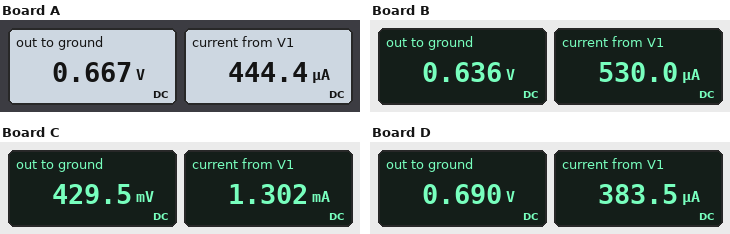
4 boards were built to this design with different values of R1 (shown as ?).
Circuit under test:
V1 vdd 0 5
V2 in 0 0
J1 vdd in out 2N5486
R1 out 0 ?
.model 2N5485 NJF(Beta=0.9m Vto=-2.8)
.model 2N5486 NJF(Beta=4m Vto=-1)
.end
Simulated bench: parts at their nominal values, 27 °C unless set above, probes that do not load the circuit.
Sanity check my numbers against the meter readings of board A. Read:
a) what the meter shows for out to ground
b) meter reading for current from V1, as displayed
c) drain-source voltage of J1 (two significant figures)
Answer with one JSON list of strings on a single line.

["0.667 V", "444.4 µA", "4.3 V"]
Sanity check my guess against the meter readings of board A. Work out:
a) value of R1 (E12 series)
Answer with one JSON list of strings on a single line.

["1.5 kΩ"]
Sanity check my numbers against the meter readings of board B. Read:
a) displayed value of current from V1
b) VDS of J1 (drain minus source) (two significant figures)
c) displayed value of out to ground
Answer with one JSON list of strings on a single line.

["530.0 µA", "4.4 V", "0.636 V"]
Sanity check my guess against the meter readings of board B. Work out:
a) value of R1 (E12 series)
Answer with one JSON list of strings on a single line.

["1.2 kΩ"]
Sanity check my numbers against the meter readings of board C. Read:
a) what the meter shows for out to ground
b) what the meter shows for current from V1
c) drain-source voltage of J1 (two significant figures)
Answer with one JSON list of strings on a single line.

["429.5 mV", "1.302 mA", "4.6 V"]
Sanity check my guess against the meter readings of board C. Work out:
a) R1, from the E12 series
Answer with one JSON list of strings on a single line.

["330 Ω"]
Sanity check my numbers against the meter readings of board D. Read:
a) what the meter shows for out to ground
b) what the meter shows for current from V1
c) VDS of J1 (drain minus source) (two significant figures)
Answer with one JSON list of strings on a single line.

["0.690 V", "383.5 µA", "4.3 V"]
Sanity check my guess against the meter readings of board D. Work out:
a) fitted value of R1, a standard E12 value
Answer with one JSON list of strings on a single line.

["1.8 kΩ"]
